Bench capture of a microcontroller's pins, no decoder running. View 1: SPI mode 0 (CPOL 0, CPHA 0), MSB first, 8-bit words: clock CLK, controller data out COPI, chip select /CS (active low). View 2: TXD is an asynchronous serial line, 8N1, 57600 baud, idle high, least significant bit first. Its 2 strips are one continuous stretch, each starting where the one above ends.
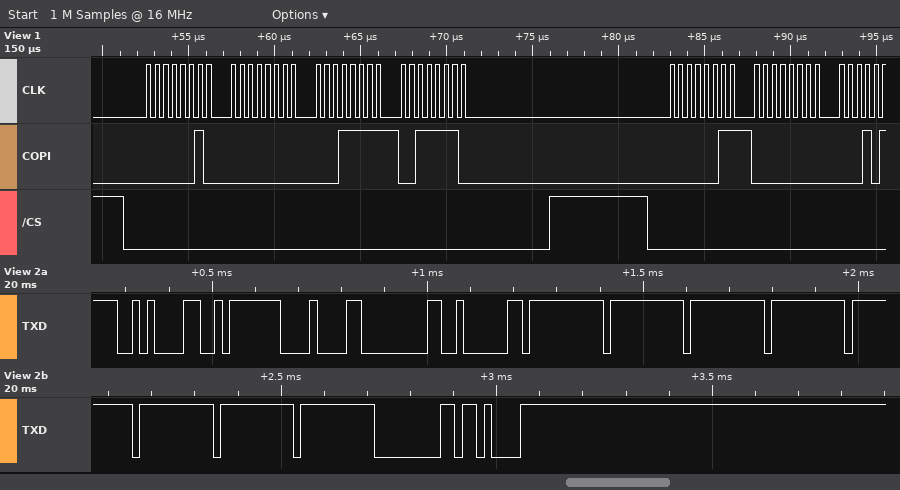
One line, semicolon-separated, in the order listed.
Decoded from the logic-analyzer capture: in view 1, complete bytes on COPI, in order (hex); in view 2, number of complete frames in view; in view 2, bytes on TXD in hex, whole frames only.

02 00 1F 3E 03 00; 15; 0A FA 08 00 02 FF FF FF FF FF FF FF FF 00 0B
